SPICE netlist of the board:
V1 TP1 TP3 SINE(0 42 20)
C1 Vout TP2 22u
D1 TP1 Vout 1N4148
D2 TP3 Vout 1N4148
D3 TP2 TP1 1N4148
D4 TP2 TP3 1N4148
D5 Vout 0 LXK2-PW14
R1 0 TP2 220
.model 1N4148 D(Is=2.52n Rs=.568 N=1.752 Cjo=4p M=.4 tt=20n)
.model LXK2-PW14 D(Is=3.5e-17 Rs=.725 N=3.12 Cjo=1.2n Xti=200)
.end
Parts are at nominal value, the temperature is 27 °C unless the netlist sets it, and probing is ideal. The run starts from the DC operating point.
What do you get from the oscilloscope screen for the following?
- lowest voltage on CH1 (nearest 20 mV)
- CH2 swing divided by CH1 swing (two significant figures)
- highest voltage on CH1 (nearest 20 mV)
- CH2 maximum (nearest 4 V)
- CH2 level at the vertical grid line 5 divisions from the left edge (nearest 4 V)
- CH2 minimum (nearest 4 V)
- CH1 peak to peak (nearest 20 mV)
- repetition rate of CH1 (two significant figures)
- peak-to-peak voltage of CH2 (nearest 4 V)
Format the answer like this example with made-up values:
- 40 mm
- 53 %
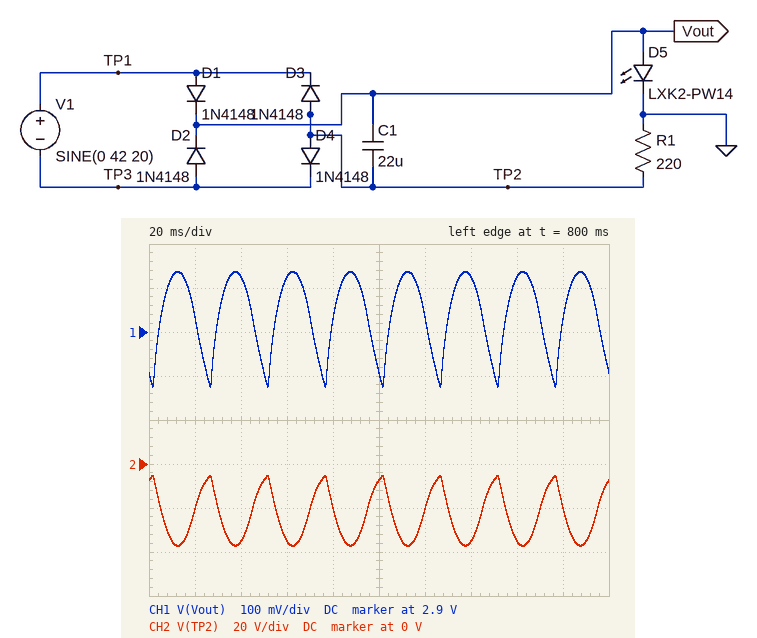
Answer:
- 2.78 V
- 120
- 3.04 V
- -4 V
- -8 V
- -36 V
- 260 mV
- 40 Hz
- 32 V
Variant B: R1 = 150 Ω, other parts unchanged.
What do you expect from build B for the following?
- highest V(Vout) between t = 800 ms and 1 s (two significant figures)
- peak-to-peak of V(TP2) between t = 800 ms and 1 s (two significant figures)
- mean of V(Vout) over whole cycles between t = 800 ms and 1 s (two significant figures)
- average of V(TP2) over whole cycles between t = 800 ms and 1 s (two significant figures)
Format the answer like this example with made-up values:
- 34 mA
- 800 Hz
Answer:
- 3.1 V
- 34 V
- 3.0 V
- -23 V
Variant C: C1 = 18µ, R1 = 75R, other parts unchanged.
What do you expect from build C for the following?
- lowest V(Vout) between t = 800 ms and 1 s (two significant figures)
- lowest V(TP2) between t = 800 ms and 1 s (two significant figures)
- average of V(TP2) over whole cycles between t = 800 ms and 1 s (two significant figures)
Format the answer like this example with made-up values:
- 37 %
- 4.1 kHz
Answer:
- 2.7 V
- -36 V
- -22 V
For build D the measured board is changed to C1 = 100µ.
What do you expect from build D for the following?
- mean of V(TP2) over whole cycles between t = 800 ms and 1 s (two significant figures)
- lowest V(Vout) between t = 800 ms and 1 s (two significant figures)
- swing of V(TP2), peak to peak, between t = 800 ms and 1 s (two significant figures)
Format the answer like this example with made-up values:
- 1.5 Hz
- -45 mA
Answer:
- -28 V
- 2.9 V
- 19 V
